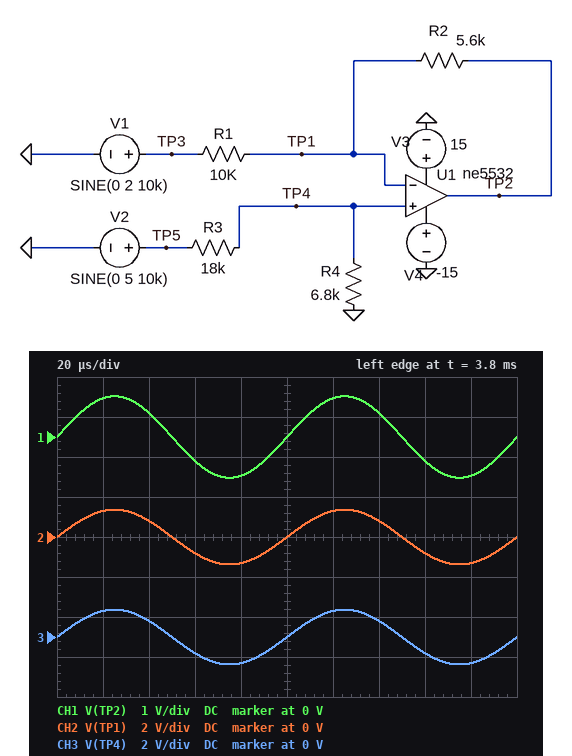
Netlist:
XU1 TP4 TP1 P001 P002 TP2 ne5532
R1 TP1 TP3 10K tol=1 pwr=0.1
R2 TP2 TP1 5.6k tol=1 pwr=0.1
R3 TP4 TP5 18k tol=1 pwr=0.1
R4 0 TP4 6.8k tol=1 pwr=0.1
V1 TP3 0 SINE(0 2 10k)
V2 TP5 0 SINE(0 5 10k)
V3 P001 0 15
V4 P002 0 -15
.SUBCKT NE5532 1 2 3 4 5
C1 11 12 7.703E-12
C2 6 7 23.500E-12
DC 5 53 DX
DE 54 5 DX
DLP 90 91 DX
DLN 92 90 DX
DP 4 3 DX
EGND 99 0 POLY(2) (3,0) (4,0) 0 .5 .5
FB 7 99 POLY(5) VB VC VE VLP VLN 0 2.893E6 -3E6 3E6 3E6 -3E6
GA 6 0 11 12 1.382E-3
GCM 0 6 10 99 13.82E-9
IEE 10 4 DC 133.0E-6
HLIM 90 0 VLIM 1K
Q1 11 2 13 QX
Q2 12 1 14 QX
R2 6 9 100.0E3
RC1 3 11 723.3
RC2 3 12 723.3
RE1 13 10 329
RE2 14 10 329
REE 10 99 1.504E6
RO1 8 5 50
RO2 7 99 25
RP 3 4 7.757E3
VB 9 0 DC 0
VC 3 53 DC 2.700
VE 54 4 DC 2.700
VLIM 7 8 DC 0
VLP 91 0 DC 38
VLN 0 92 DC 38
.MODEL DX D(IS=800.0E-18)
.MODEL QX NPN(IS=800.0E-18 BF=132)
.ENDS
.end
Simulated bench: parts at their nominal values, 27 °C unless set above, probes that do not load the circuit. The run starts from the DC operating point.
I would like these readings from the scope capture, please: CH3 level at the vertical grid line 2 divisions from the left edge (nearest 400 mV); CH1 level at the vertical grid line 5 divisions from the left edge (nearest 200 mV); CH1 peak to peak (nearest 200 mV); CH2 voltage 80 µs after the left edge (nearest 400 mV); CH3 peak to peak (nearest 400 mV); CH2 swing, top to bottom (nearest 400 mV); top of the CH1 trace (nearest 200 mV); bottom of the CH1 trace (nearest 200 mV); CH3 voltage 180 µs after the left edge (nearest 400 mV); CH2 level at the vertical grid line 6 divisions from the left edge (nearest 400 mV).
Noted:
800 mV
0 V
2.0 V
-1.2 V
2.8 V
2.8 V
1.0 V
-1.0 V
-1.2 V
1.2 V
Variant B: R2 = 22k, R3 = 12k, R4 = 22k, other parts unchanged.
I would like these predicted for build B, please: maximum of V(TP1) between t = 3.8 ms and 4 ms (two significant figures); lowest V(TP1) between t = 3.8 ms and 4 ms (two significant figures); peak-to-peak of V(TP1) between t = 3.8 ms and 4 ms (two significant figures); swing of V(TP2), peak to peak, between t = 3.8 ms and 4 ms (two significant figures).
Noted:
3.2 V
-3.2 V
6.5 V
12 V
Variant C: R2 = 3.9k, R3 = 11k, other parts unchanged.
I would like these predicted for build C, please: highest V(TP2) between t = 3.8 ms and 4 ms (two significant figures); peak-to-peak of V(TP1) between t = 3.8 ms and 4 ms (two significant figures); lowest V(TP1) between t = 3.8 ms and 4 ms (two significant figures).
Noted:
1.9 V
3.8 V
-1.9 V
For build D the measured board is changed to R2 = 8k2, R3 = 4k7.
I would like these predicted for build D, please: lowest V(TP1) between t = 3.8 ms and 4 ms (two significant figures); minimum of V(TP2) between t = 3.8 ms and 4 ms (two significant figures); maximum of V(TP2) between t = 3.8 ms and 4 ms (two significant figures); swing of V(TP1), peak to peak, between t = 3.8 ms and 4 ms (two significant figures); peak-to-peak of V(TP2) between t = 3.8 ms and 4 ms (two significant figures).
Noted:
-3.0 V
-3.7 V
3.7 V
5.9 V
7.5 V
